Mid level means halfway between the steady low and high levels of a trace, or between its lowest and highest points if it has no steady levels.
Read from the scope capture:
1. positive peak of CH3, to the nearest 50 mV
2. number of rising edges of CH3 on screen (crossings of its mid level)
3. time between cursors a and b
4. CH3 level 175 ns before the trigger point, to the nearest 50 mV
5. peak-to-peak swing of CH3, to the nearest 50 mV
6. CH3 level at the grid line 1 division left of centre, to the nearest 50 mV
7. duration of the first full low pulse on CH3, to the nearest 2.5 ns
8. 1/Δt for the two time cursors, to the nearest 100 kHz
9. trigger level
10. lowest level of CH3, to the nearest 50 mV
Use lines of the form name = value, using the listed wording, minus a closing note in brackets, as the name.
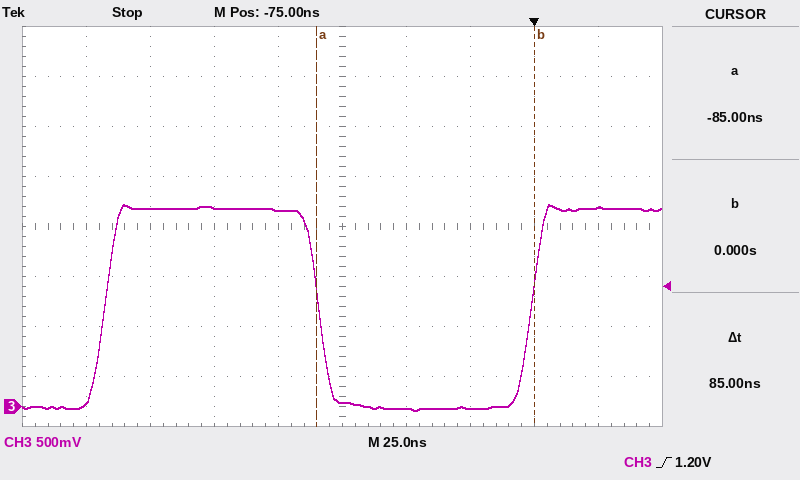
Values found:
positive peak of CH3, to the nearest 50 mV = 2.00 V
number of rising edges of CH3 on screen = 2
time between cursors a and b = 85 ns
CH3 level 175 ns before the trigger point, to the nearest 50 mV = 50 mV
peak-to-peak swing of CH3, to the nearest 50 mV = 2.05 V
CH3 level at the grid line 1 division left of centre, to the nearest 50 mV = 1.95 V
duration of the first full low pulse on CH3, to the nearest 2.5 ns = 82.5 ns
1/Δt for the two time cursors, to the nearest 100 kHz = 11.8 MHz
trigger level = 1.20 V
lowest level of CH3, to the nearest 50 mV = -50 mV
